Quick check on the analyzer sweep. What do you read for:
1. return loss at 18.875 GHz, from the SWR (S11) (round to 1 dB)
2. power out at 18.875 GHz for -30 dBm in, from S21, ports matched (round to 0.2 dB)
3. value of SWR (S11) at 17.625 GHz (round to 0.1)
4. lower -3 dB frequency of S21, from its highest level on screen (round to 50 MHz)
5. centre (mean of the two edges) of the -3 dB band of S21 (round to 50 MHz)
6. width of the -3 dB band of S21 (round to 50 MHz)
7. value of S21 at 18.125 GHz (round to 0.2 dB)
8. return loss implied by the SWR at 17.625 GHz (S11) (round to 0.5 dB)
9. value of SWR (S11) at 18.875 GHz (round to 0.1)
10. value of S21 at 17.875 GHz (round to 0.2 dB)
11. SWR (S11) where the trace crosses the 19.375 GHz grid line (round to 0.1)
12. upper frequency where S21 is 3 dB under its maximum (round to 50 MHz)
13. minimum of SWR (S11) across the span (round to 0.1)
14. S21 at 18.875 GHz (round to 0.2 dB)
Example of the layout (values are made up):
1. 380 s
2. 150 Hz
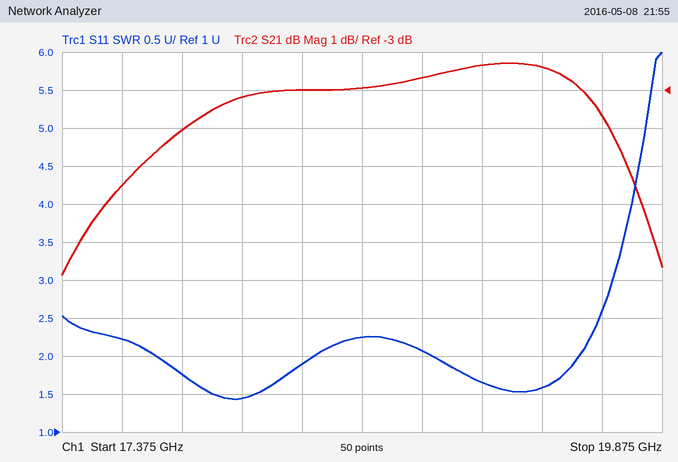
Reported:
1. 9 dB
2. -32.6 dBm
3. 2.2
4. 17.65 GHz
5. 18.70 GHz
6. 2.10 GHz
7. -3.2 dB
8. 8.5 dB
9. 2.1
10. -4.0 dB
11. 1.6
12. 19.75 GHz
13. 1.4
14. -2.6 dB
